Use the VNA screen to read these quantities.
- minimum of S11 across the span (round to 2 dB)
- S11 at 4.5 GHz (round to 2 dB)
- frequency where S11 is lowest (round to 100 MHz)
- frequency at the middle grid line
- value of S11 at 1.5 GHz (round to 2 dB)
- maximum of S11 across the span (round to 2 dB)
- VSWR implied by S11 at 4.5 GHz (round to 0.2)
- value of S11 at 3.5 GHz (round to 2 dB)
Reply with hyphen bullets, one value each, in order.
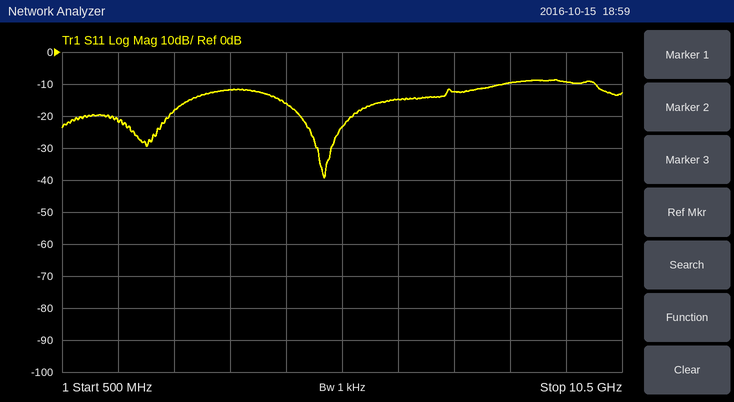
- -40 dB
- -16 dB
- 5.2 GHz
- 5.5 GHz
- -22 dB
- -8 dB
- 1.4
- -12 dB
